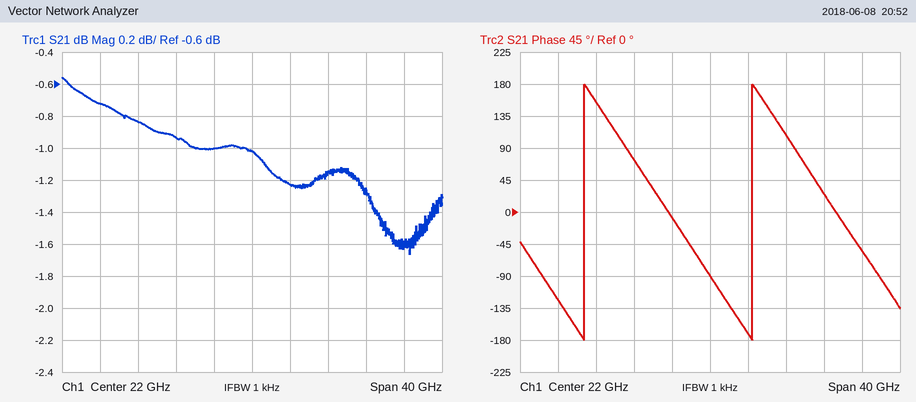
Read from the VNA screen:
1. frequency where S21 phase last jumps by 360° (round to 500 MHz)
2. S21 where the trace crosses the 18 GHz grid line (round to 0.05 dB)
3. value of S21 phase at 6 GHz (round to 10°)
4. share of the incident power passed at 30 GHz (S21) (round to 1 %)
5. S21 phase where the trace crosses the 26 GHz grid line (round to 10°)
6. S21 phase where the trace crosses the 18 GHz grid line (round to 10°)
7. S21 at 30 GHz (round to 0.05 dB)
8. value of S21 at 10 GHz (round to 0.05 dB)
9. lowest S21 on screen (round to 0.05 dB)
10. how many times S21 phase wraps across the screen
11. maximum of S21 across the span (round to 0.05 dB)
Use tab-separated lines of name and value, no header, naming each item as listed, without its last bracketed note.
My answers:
frequency where S21 phase last jumps by 360°	26.5 GHz
S21 where the trace crosses the 18 GHz grid line	-1.00 dB
value of S21 phase at 6 GHz	-120°
share of the incident power passed at 30 GHz (S21)	77 %
S21 phase where the trace crosses the 26 GHz grid line	-170°
S21 phase where the trace crosses the 18 GHz grid line	-10°
S21 at 30 GHz	-1.15 dB
value of S21 at 10 GHz	-0.85 dB
lowest S21 on screen	-1.65 dB
how many times S21 phase wraps across the screen	2
maximum of S21 across the span	-0.55 dB
